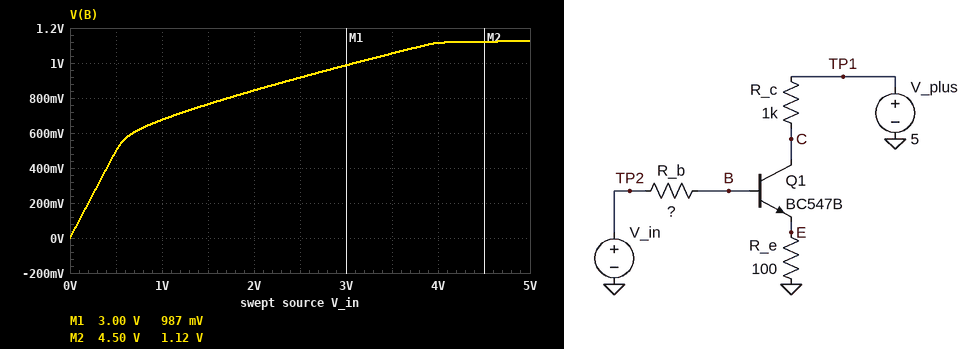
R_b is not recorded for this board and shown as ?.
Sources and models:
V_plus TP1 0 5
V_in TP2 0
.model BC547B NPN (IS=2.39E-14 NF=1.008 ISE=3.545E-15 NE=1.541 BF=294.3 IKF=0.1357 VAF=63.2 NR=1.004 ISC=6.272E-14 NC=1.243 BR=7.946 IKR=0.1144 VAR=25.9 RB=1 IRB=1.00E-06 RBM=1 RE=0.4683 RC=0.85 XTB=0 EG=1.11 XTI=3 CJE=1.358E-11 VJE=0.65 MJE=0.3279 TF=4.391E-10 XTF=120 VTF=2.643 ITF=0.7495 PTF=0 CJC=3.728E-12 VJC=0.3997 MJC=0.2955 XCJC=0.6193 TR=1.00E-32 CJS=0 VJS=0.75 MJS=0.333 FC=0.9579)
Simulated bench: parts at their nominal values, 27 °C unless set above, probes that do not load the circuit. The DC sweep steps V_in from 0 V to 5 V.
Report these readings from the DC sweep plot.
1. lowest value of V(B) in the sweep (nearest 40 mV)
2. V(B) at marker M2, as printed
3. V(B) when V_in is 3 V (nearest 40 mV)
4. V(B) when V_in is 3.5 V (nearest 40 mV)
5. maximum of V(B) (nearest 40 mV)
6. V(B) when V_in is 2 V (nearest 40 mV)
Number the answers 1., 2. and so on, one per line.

1. 0 V
2. 1.12 V
3. 1.00 V
4. 1.04 V
5. 1.12 V
6. 840 mV
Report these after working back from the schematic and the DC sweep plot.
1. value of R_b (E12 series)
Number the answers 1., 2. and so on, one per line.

1. 180 kΩ
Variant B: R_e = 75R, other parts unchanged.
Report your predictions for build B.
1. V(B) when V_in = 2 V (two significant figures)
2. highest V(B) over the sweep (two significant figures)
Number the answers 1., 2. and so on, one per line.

1. 800 mV
2. 1.0 V
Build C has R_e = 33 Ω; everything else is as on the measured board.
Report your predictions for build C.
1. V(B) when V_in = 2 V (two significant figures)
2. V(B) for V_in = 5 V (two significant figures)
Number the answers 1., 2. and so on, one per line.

1. 730 mV
2. 840 mV
